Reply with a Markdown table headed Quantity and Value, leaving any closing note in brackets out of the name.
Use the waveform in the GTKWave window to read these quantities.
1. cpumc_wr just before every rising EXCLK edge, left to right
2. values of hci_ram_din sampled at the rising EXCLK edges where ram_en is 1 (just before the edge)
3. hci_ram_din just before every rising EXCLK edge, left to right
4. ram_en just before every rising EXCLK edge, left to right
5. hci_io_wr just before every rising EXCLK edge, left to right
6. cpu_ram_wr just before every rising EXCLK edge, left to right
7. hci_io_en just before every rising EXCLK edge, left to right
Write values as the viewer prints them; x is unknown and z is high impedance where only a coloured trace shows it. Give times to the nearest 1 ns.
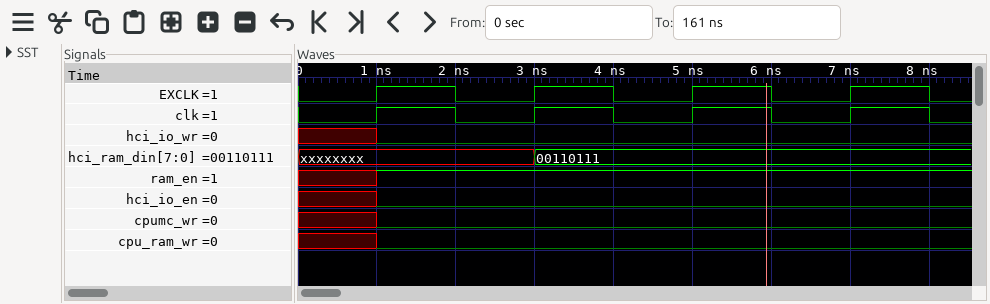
| Quantity | Value |
|---|---|
| cpumc_wr just before every rising EXCLK edge, left to right | x 0 0 0 |
| values of hci_ram_din sampled at the rising EXCLK edges where ram_en is 1 | xxxxxxxx, 00110111, 00110111 |
| hci_ram_din just before every rising EXCLK edge, left to right | xxxxxxxx, xxxxxxxx, 00110111, 00110111 |
| ram_en just before every rising EXCLK edge, left to right | x 1 1 1 |
| hci_io_wr just before every rising EXCLK edge, left to right | x 0 0 0 |
| cpu_ram_wr just before every rising EXCLK edge, left to right | x 0 0 0 |
| hci_io_en just before every rising EXCLK edge, left to right | x 0 0 0 |
